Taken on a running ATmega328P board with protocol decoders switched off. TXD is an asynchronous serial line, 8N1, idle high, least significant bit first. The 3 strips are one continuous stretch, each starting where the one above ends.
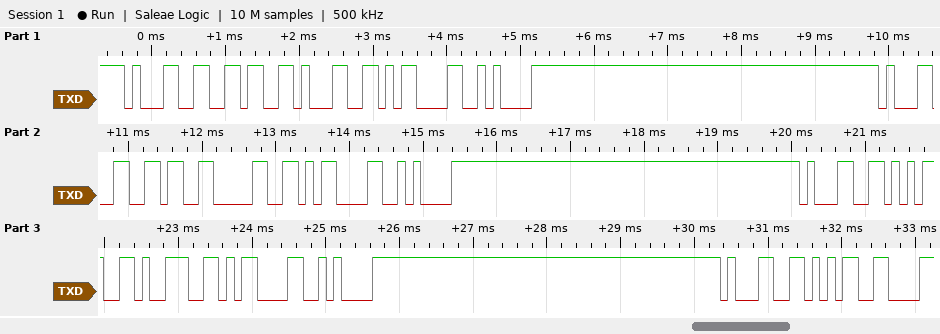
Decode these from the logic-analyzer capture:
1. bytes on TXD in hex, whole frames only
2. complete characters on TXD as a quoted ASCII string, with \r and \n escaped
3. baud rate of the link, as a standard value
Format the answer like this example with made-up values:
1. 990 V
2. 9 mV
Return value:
1. 31 36 31 0D 0A 31 36 30 0D 0A 31 35 39 0D 0A 31 35
2. "161\r\n160\r\n159\r\n15"
3. 9600 baud
